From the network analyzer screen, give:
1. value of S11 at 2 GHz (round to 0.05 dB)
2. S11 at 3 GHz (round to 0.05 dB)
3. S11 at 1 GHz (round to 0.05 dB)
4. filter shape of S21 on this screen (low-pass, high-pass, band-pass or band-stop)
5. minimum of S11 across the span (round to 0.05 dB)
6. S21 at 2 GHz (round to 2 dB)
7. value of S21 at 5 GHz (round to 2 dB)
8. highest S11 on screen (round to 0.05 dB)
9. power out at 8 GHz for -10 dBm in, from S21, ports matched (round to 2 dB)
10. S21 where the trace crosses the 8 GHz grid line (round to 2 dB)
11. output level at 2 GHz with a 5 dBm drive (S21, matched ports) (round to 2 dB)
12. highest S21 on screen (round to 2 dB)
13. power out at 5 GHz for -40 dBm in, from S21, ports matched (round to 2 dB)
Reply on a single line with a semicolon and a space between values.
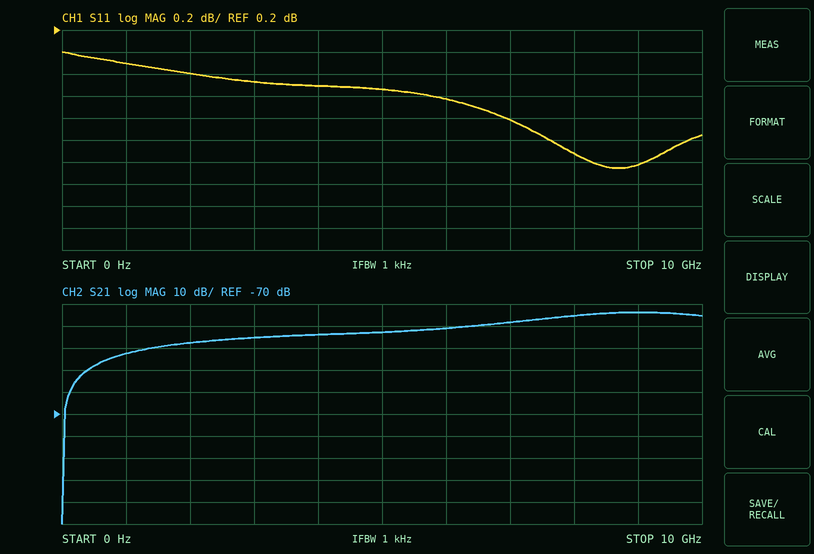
-0.20 dB; -0.25 dB; -0.10 dB; high-pass; -1.05 dB; -38 dB; -32 dB; 0.00 dB; -36 dBm; -26 dB; -32 dBm; -24 dB; -72 dBm
